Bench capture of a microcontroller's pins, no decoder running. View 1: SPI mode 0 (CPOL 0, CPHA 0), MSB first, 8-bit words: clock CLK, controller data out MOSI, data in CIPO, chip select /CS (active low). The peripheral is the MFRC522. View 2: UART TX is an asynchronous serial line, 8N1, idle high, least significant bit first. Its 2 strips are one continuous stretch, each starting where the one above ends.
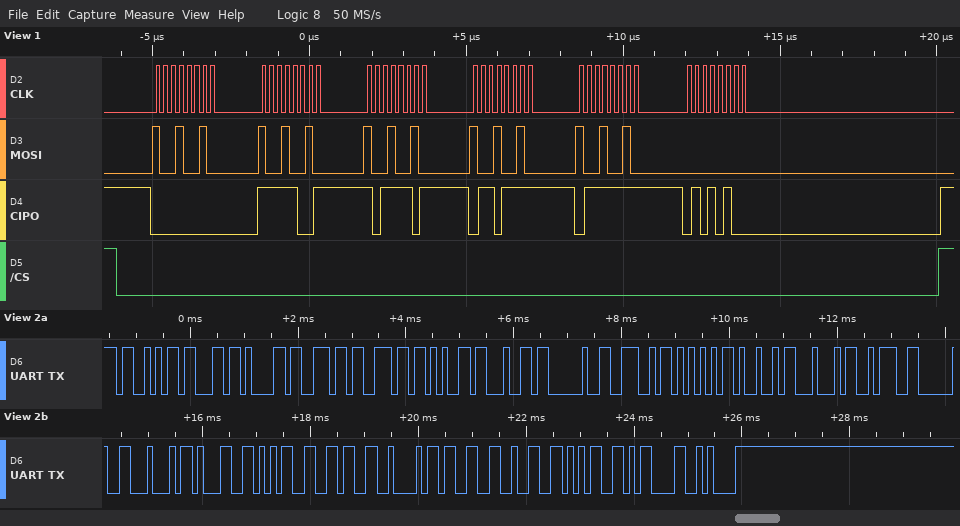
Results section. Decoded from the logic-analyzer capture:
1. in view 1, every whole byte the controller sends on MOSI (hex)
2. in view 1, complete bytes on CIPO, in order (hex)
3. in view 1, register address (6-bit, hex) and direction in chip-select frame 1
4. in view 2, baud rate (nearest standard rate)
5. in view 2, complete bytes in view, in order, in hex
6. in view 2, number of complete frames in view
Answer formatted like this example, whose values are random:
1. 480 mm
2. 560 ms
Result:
1. 92 92 92 92 92 00
2. 00 F9 BD 6F 7F 54
3. 0x09 read
4. 9600 baud
5. 53 63 61 6E 6E 65 64 20 4E 55 49 44 3A 20 44 31 35 36 42 33 32 35 0D 0A
6. 24
